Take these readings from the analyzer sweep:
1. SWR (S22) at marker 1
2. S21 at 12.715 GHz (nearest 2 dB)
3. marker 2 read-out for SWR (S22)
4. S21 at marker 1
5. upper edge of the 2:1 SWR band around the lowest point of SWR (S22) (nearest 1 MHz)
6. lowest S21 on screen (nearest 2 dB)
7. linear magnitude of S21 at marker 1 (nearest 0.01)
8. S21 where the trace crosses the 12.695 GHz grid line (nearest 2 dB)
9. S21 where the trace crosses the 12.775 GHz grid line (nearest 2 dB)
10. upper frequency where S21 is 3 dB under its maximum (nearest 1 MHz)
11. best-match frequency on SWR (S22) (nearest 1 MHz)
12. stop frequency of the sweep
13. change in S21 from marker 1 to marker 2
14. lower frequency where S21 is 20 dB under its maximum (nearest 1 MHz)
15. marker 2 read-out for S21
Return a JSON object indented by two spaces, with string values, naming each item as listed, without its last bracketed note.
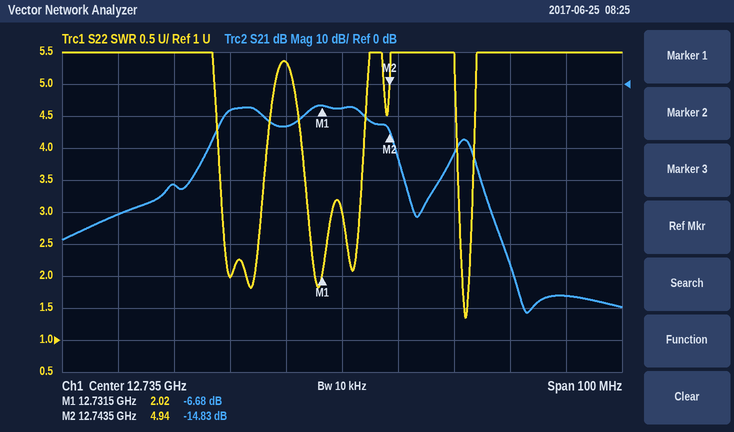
{
  "SWR (S22) at marker 1": "2.02",
  "S21 at 12.715 GHz": "-8 dB",
  "marker 2 read-out for SWR": "4.94",
  "S21 at marker 1": "-6.68 dB",
  "upper edge of the 2:1 SWR band around the lowest point of SWR (S22)": "12.758 GHz",
  "lowest S21 on screen": "-72 dB",
  "linear magnitude of S21 at marker 1": "0.46",
  "S21 where the trace crosses the 12.695 GHz grid line": "-40 dB",
  "S21 where the trace crosses the 12.775 GHz grid line": "-66 dB",
  "upper frequency where S21 is 3 dB under its maximum": "12.739 GHz",
  "best-match frequency on SWR (S22)": "12.757 GHz",
  "stop frequency of the sweep": "12.785 GHz",
  "change in S21 from marker 1 to marker 2": "-8.15 dB",
  "lower frequency where S21 is 20 dB under its maximum": "12.709 GHz",
  "marker 2 read-out for S21": "-14.83 dB"
}
